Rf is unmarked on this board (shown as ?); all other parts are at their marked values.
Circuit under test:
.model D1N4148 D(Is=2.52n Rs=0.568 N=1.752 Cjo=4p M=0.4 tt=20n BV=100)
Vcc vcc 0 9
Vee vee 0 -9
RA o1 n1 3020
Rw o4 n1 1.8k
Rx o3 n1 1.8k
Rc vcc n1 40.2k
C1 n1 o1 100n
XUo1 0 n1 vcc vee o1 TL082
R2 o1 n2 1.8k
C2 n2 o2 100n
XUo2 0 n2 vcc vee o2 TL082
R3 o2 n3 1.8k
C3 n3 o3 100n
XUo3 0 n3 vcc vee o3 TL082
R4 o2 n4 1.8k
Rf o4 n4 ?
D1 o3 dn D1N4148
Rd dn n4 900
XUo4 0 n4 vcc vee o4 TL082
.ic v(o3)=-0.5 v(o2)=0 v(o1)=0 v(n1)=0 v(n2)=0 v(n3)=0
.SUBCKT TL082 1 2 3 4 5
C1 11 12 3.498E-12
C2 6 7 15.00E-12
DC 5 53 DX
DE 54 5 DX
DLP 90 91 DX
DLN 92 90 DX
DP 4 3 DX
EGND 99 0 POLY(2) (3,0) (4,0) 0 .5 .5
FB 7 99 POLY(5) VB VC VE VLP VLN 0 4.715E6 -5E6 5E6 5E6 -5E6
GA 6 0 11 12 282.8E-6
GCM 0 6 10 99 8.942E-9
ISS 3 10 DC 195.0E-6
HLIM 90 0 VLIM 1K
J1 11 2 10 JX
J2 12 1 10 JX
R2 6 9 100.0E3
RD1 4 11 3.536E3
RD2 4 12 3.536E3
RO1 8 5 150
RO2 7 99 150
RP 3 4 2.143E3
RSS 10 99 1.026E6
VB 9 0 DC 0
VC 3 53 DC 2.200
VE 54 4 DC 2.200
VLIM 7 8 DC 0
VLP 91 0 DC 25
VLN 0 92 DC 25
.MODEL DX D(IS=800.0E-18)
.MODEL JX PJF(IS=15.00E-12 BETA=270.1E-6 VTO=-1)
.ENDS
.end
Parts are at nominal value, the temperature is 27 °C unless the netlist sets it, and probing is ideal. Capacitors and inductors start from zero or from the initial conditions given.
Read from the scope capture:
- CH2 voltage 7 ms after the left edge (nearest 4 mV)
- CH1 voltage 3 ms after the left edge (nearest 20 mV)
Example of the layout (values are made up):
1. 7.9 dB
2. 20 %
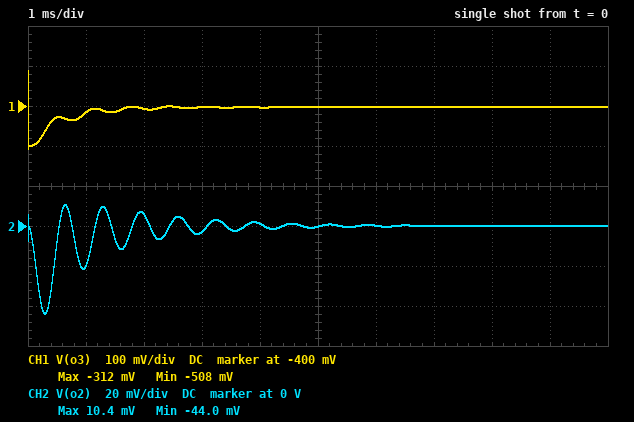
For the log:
1. 0 V
2. -400 mV
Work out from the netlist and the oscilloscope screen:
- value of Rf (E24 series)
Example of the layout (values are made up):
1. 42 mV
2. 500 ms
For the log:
1. 5.6 kΩ
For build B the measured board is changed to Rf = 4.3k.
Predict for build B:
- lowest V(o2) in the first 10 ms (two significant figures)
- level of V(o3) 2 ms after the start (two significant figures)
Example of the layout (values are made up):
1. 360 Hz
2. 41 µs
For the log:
1. -53 mV
2. -390 mV
